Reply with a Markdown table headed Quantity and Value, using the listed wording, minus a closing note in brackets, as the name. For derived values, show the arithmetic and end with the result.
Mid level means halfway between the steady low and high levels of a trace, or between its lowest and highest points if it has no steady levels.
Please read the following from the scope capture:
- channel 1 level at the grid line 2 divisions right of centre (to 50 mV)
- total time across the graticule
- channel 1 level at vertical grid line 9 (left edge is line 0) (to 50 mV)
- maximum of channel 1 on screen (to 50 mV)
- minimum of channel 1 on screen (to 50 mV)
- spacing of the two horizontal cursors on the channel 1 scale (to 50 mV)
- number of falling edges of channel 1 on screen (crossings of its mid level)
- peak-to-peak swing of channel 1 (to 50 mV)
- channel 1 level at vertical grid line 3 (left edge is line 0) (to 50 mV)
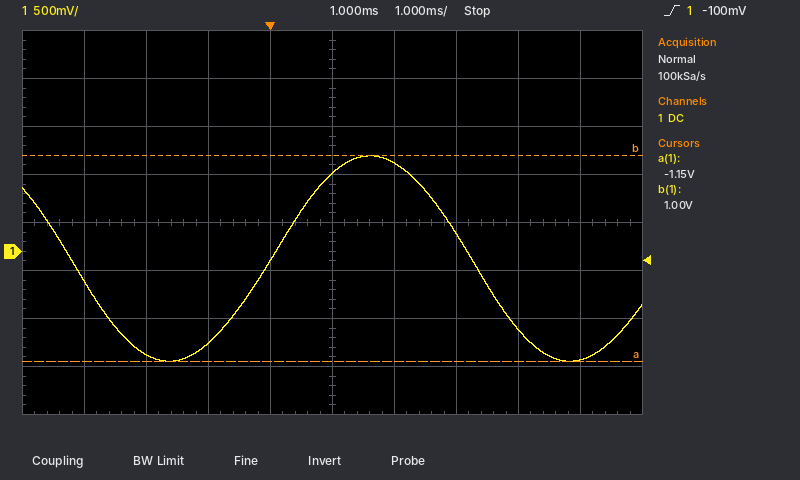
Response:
| Quantity | Value |
|---|---|
| channel 1 level at the grid line 2 divisions right of centre | 200 mV |
| total time across the graticule | 10 ms |
| channel 1 level at vertical grid line 9 (left edge is line 0) | -1.15 V |
| maximum of channel 1 on screen | 1.00 V |
| minimum of channel 1 on screen | -1.15 V |
| spacing of the two horizontal cursors on the channel 1 scale | 2.15 V |
| number of falling edges of channel 1 on screen | 2 |
| peak-to-peak swing of channel 1 | 1.00 V − (-1.15 V) = 2.15 V |
| channel 1 level at vertical grid line 3 (left edge is line 0) | -950 mV |
